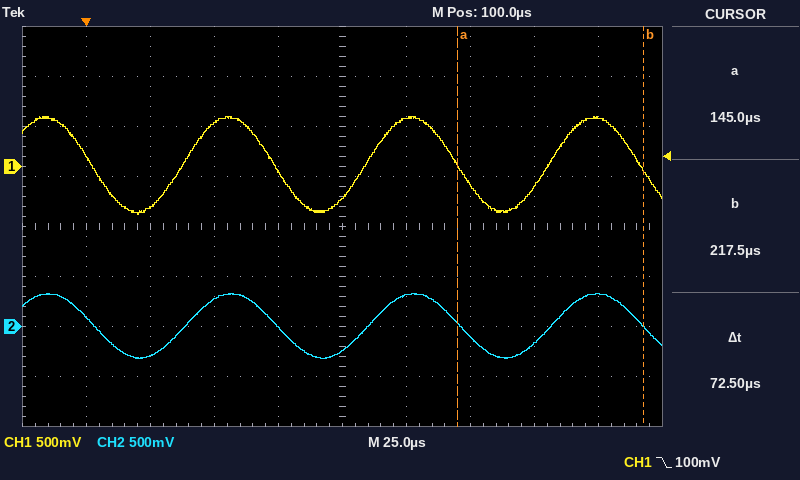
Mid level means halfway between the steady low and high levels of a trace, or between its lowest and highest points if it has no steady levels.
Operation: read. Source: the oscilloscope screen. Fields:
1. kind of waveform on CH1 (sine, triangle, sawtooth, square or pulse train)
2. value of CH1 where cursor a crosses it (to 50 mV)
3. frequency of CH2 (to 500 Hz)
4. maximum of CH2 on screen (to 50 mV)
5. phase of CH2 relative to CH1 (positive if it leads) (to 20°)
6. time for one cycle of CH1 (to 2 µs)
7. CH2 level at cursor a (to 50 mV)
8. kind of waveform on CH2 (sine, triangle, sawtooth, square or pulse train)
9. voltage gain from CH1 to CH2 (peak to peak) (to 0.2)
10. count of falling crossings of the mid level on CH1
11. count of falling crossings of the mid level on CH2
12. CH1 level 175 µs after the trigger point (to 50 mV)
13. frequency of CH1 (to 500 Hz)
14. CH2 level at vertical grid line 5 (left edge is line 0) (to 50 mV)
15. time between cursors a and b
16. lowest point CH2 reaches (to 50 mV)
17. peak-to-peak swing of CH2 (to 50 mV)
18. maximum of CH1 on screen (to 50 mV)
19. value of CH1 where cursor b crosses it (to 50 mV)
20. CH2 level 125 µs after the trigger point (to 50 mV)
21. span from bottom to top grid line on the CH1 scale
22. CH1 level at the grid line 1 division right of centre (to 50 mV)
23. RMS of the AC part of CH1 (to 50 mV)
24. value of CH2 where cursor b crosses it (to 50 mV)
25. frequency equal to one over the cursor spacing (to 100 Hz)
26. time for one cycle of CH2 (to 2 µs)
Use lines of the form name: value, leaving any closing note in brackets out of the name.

kind of waveform on CH1: sine
value of CH1 where cursor a crosses it: 0 mV
frequency of CH2: 14.0 kHz
maximum of CH2 on screen: 350 mV
phase of CH2 relative to CH1 (positive if it leads): 0°
time for one cycle of CH1: 72 µs
CH2 level at cursor a: 50 mV
kind of waveform on CH2: sine
voltage gain from CH1 to CH2 (peak to peak): 0.6
count of falling crossings of the mid level on CH1: 4
count of falling crossings of the mid level on CH2: 4
CH1 level 175 µs after the trigger point: -200 mV
frequency of CH1: 14.0 kHz
CH2 level at vertical grid line 5 (left edge is line 0): -250 mV
time between cursors a and b: 72.5 µs
lowest point CH2 reaches: -300 mV
peak-to-peak swing of CH2: 650 mV
maximum of CH1 on screen: 500 mV
value of CH1 where cursor b crosses it: -50 mV
CH2 level 125 µs after the trigger point: 300 mV
span from bottom to top grid line on the CH1 scale: 4 V
CH1 level at the grid line 1 division right of centre: 500 mV
RMS of the AC part of CH1: 350 mV
value of CH2 where cursor b crosses it: 0 mV
frequency equal to one over the cursor spacing: 13.8 kHz
time for one cycle of CH2: 72 µs
